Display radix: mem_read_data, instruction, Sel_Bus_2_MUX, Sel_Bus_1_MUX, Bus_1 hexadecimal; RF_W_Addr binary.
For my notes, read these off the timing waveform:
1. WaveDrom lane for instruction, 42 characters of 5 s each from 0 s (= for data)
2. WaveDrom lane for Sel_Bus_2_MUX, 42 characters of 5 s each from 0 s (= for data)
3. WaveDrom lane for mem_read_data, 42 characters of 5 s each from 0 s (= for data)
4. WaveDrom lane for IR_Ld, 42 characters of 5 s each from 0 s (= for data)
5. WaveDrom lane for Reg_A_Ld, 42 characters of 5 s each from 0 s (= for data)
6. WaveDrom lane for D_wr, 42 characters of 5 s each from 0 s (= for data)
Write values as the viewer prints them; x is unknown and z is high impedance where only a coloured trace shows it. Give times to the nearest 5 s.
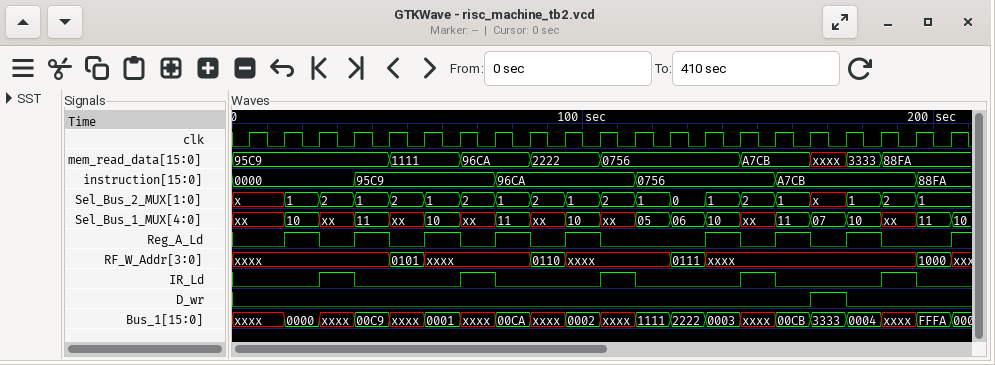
{name: 'instruction', wave: '=......=.......=.......=.......=.......=..', data: '0000 95C9 96CA 0756 A7CB 88FA'}
{name: 'Sel_Bus_2_MUX', wave: 'x..=.=.=.=.=.=.=.=.=.=.=.=.=.=.=.x.=.=.=..', data: '1 2 1 2 1 2 1 2 1 2 1 0 1 2 1 1 2 1'}
{name: 'mem_read_data', wave: '=........=...=...=...=.......=...x.=.=....', data: '95C9 1111 96CA 2222 0756 A7CB 3333 88FA'}
{name: 'IR_Ld', wave: '0....1.0.....1.0.....1.0.....1.0.....1.0..'}
{name: 'Reg_A_Ld', wave: '0..1.0.1.0.1.0.1.0.1.0.....1.0.1.0.1.0...1'}
{name: 'D_wr', wave: '0................................1.0......'}
